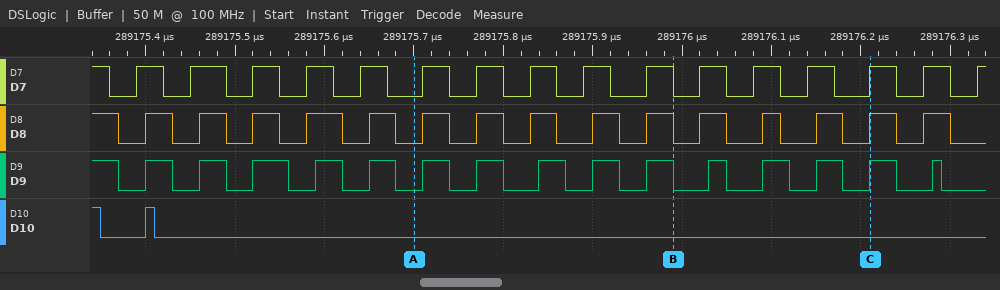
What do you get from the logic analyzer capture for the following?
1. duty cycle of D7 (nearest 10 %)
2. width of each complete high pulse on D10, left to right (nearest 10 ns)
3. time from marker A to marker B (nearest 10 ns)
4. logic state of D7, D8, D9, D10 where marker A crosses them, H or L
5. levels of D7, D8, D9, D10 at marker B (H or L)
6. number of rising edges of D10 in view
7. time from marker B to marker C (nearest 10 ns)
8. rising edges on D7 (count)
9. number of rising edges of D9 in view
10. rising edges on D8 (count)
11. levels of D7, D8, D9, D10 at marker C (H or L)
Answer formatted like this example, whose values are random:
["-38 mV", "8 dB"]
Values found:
["50 %", "10 ns", "290 ns", "D7=L, D8=L, D9=L, D10=L", "D7=L, D8=L, D9=L, D10=L", "1", "220 ns", "16", "15", "15", "D7=H, D8=H, D9=H, D10=L"]
